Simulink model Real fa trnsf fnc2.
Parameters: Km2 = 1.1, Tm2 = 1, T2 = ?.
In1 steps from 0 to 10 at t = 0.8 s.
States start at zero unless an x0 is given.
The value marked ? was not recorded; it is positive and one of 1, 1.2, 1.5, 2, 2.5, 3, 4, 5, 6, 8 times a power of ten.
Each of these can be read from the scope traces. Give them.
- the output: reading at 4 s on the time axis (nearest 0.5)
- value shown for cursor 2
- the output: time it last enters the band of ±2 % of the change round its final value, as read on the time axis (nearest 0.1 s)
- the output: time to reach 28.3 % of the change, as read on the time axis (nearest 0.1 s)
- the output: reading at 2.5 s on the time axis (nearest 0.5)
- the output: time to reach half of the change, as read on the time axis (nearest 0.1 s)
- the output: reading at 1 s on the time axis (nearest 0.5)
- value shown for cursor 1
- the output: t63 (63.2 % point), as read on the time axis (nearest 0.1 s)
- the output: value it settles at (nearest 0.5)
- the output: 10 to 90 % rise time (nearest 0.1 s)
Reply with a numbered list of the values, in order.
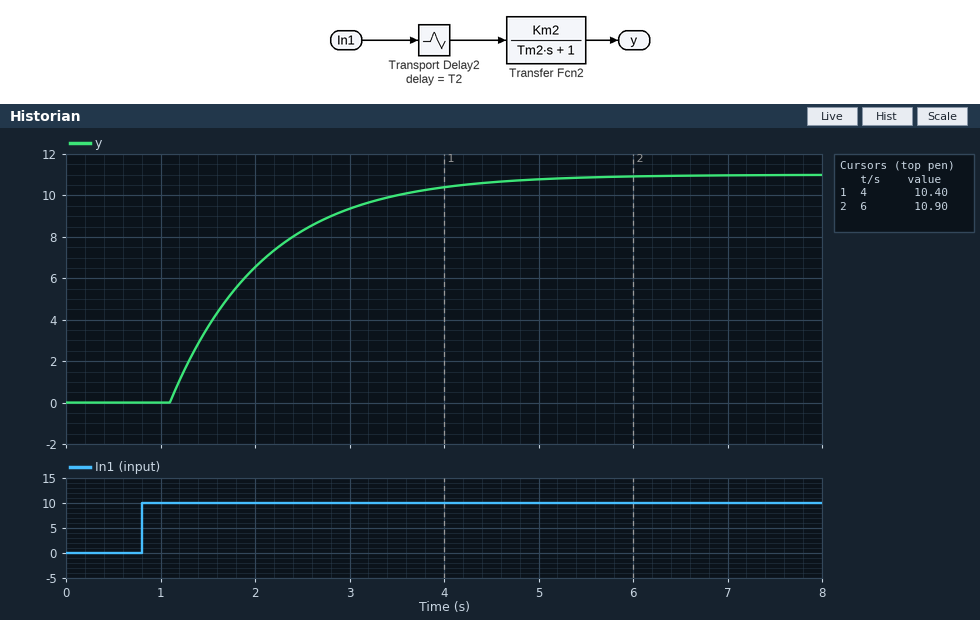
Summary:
1. 10.5
2. 10.90
3. 5.0 s
4. 1.4 s
5. 8.5
6. 1.8 s
7. 0.0
8. 10.40
9. 2.1 s
10. 11.0
11. 2.2 s
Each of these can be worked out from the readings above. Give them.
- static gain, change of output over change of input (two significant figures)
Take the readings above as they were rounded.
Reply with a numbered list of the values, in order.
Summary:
1. 1.1
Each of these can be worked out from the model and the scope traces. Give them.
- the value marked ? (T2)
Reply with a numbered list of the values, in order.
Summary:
1. 0.3
